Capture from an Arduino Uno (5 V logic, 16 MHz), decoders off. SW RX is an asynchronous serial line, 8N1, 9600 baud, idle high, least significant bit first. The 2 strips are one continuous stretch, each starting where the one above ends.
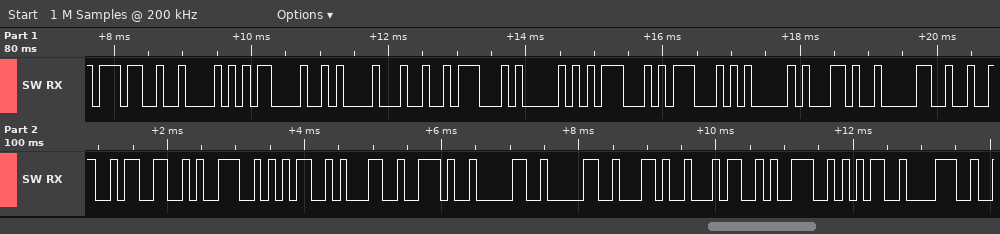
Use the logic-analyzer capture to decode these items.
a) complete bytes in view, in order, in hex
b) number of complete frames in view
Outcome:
37 42 0D 0A 24 47 50 47 47 41 2C 30 32 33 39 35 31 2E 30 30 2C 34 39 35 38
25
